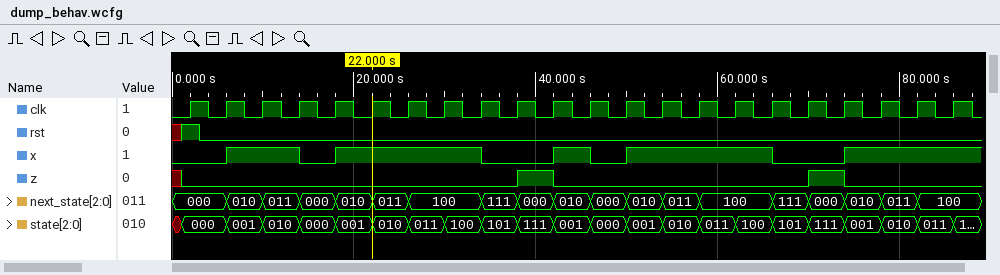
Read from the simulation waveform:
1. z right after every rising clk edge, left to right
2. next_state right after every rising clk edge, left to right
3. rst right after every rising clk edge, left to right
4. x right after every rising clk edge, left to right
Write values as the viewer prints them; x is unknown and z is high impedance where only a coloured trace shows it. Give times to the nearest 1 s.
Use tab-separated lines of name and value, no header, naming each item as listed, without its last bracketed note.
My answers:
z right after every rising clk edge, left to right	0 0 0 0 0 0 0 0 0 1 0 0 0 0 0 0 0 1 0 0 0 0
next_state right after every rising clk edge, left to right	000, 010, 011, 000, 010, 011, 100, 100, 111, 000, 010, 000, 010, 011, 100, 100, 111, 000, 010, 011, 100, 100
rst right after every rising clk edge, left to right	1 0 0 0 0 0 0 0 0 0 0 0 0 0 0 0 0 0 0 0 0 0
x right after every rising clk edge, left to right	0 1 1 0 1 1 1 1 0 0 1 0 1 1 1 1 0 0 1 1 1 1
